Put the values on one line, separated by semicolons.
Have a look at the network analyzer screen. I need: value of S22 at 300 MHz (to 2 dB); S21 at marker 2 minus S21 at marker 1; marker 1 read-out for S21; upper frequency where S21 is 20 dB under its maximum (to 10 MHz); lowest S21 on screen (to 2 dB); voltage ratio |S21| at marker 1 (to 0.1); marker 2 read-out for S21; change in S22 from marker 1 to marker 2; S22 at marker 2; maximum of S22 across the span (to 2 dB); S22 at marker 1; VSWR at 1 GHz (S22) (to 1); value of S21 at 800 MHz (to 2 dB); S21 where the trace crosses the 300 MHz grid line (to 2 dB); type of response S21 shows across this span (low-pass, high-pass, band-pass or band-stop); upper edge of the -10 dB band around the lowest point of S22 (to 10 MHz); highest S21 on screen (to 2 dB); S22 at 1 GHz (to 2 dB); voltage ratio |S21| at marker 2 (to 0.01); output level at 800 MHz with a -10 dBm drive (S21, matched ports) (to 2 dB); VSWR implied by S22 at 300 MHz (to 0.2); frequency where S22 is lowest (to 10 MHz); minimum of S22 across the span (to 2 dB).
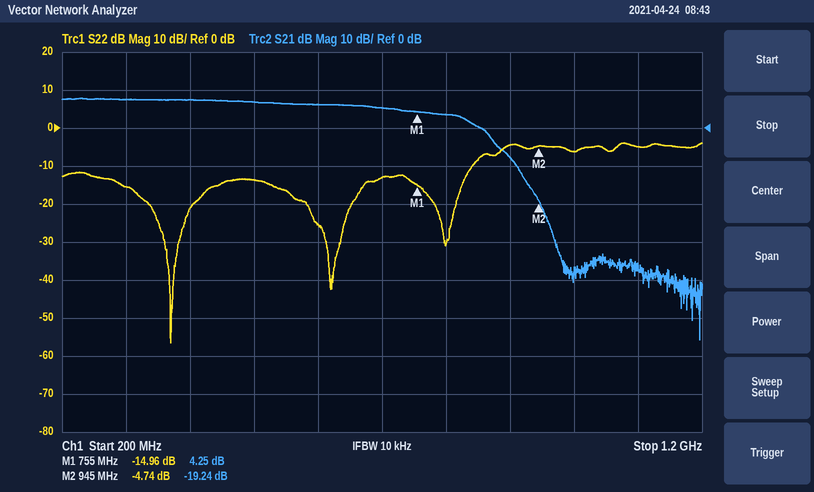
-16 dB; -23.49 dB; 4.25 dB; 920 MHz; -56 dB; 1.6; -19.24 dB; 10.22 dB; -4.74 dB; -4 dB; -14.96 dB; 3; 4 dB; 8 dB; low-pass; 840 MHz; 8 dB; -6 dB; 0.11; -6 dBm; 1.4; 370 MHz; -56 dB
